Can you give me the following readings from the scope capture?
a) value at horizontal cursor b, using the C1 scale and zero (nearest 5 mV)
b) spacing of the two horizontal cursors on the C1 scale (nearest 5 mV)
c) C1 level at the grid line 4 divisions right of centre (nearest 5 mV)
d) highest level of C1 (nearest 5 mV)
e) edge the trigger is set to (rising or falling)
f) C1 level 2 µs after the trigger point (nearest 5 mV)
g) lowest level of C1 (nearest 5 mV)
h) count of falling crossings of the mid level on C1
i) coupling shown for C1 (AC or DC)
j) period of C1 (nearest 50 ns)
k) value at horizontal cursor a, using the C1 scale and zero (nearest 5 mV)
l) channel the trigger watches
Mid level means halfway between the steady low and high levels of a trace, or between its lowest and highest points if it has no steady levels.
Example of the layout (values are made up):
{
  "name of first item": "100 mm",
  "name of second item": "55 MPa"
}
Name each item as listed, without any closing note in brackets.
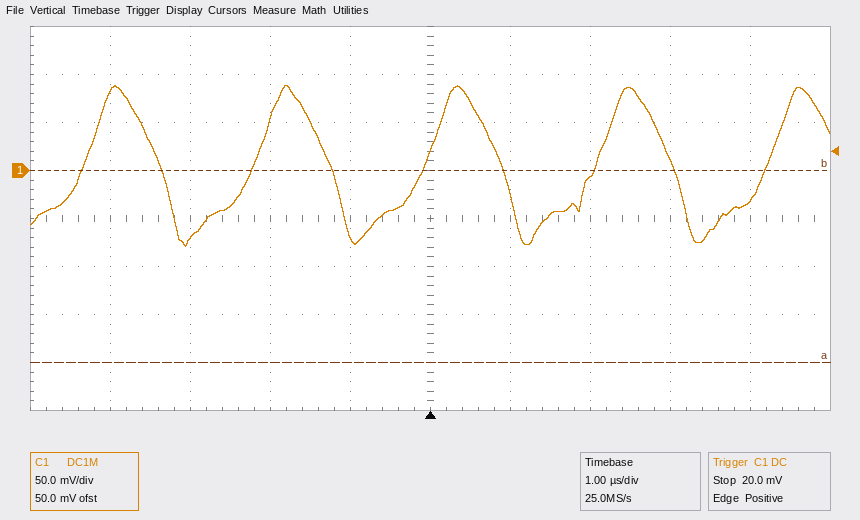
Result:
{
  "value at horizontal cursor b, using the C1 scale and zero": "0 mV",
  "spacing of the two horizontal cursors on the C1 scale": "200 mV",
  "C1 level at the grid line 4 divisions right of centre": "-30 mV",
  "highest level of C1": "90 mV",
  "edge the trigger is set to": "rising",
  "C1 level 2 µs after the trigger point": "-5 mV",
  "lowest level of C1": "-80 mV",
  "count of falling crossings of the mid level on C1": "4",
  "coupling shown for C1": "DC",
  "period of C1": "2.15 µs",
  "value at horizontal cursor a, using the C1 scale and zero": "-200 mV",
  "channel the trigger watches": "C1"
}
